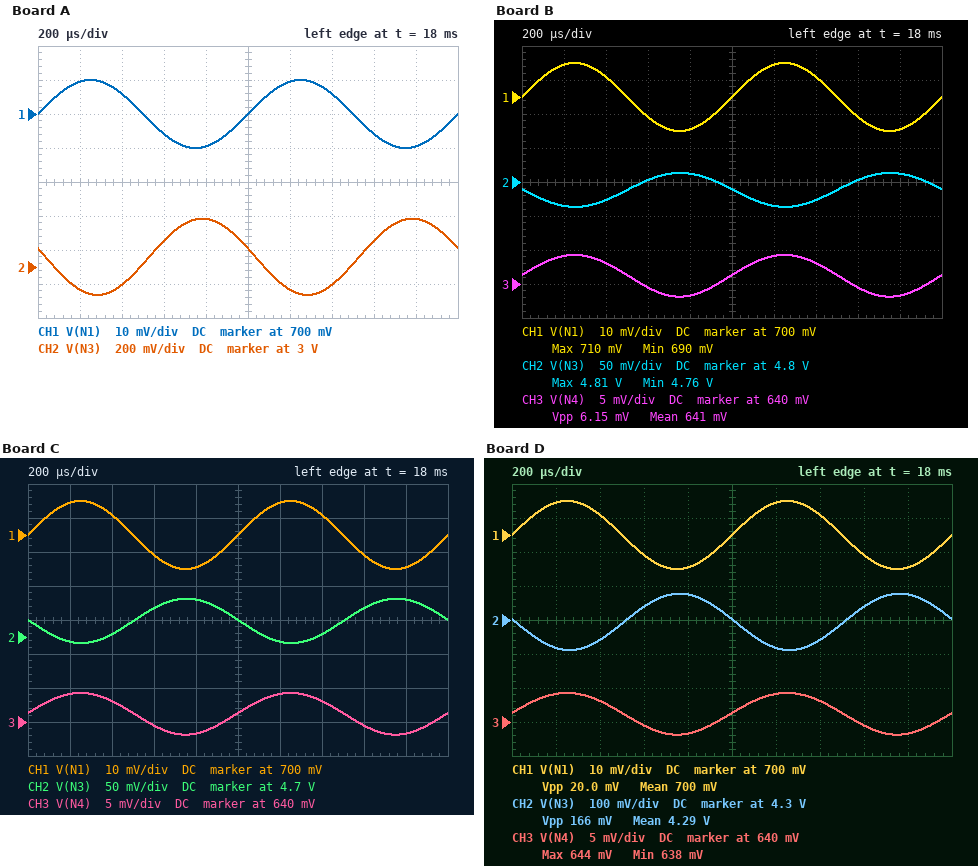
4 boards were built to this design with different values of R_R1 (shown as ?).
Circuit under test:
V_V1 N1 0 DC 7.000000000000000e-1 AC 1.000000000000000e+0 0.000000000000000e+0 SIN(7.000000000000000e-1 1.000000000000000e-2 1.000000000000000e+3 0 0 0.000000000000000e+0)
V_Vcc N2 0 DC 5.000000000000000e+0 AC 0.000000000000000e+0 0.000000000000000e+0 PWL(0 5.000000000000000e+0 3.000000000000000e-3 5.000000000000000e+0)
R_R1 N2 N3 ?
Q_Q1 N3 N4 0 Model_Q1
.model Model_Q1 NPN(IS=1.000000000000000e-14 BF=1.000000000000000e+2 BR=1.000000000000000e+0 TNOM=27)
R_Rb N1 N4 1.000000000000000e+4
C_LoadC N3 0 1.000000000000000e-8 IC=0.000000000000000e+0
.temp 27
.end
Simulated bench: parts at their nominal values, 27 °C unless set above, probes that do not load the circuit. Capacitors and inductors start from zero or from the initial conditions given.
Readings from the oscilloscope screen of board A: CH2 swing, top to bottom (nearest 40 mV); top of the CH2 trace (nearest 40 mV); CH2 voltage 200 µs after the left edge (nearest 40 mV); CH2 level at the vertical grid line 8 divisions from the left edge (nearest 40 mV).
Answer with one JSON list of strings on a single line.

["440 mV", "3.28 V", "2.88 V", "3.16 V"]
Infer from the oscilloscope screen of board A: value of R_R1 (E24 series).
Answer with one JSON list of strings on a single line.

["3.3 kΩ"]
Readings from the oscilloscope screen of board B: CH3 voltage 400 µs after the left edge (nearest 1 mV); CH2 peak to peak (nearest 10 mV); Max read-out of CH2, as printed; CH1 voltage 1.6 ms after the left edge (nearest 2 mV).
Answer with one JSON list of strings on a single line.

["643 mV", "50 mV", "4.81 V", "694 mV"]
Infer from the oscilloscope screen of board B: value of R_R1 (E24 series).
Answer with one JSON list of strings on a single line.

["360 Ω"]
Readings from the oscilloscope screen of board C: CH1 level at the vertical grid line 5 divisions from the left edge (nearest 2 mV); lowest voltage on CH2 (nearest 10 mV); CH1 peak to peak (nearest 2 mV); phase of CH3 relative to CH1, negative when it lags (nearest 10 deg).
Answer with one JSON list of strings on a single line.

["700 mV", "4.69 V", "20 mV", "0 deg"]
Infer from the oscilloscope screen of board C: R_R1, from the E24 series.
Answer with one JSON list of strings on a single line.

["470 Ω"]
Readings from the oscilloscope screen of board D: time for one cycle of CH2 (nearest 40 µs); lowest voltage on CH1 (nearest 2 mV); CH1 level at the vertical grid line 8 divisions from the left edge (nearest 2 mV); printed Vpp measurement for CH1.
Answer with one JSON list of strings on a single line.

["1.00 ms", "690 mV", "694 mV", "20.0 mV"]
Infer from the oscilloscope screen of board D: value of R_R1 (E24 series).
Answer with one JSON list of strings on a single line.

["1.2 kΩ"]
